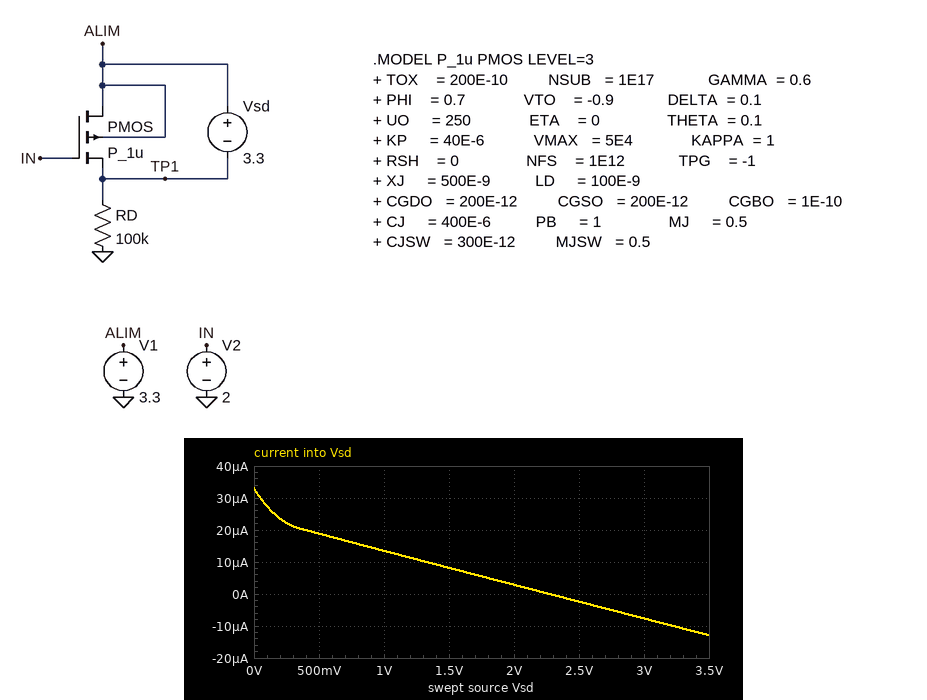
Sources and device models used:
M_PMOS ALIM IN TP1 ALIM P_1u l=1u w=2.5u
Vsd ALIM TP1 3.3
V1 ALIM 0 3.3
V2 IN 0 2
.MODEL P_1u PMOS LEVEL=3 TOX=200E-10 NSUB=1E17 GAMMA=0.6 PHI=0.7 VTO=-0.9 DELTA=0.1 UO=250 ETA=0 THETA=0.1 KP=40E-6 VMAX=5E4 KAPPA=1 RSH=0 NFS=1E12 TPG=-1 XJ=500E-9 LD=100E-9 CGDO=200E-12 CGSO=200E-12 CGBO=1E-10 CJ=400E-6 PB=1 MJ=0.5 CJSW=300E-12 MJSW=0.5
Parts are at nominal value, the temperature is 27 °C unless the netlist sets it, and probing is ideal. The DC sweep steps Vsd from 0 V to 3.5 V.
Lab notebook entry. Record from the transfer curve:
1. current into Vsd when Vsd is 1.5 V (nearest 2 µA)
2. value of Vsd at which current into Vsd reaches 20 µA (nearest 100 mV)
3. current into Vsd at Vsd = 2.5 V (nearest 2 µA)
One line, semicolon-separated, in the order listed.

8 µA; 400 mV; -2 µA
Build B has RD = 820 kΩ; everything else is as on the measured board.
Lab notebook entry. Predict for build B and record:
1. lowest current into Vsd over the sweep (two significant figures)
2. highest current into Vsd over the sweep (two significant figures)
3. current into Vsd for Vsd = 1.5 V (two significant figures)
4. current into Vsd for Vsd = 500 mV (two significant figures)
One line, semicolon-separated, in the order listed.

-11 µA; 4.0 µA; -7.6 µA; -5.7 µA
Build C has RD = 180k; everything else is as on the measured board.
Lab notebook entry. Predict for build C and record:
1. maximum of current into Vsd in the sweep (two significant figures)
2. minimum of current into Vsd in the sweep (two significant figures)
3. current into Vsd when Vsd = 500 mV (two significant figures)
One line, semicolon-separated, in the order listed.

18 µA; -12 µA; 6.4 µA
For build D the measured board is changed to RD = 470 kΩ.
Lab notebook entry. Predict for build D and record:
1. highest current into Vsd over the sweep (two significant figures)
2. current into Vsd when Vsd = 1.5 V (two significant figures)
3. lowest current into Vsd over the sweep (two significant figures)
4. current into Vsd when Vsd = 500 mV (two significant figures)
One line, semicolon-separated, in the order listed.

7.0 µA; -6.0 µA; -11 µA; -3.2 µA
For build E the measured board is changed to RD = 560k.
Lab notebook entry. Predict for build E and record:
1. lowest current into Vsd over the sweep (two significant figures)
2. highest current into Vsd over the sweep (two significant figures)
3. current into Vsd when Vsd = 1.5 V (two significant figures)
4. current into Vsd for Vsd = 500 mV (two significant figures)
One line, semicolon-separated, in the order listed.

-11 µA; 5.9 µA; -6.6 µA; -4.1 µA
